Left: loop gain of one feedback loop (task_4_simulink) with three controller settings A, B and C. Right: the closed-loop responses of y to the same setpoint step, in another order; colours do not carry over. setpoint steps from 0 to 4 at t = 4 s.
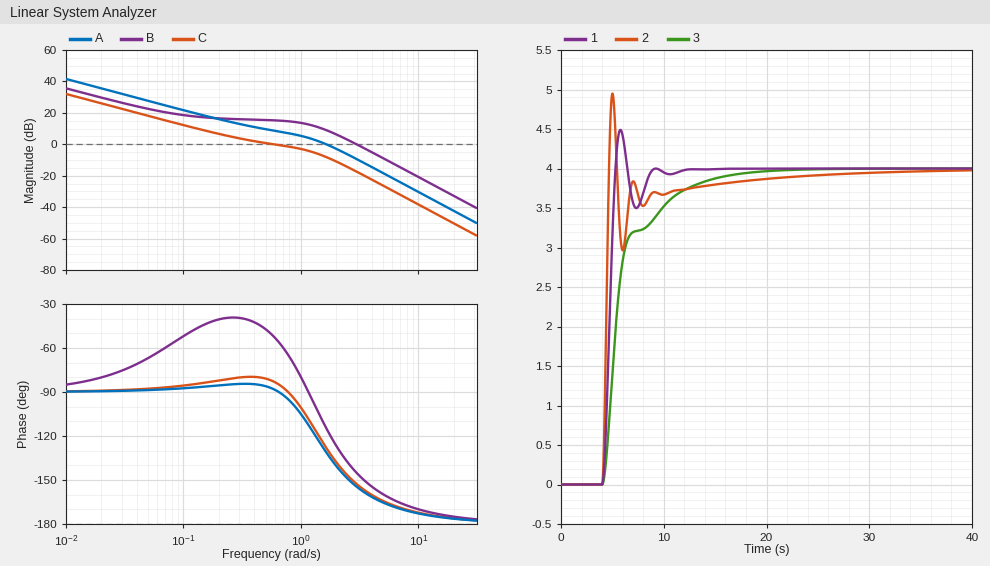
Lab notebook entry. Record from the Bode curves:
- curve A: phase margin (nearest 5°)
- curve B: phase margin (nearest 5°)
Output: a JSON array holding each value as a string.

["50°", "35°"]
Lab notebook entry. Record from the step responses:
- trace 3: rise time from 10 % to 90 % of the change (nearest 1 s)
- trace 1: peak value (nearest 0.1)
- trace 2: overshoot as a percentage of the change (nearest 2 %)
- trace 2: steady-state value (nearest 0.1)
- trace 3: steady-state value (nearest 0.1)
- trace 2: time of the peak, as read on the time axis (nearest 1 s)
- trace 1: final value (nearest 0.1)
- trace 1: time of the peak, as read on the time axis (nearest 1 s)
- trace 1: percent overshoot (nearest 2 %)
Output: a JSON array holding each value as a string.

["6 s", "4.5", "24 %", "4.0", "4.0", "5 s", "4.0", "6 s", "12 %"]
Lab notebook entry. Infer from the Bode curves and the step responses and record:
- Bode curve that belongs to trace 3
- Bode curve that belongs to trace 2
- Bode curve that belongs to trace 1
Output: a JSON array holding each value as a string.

["C", "B", "A"]
